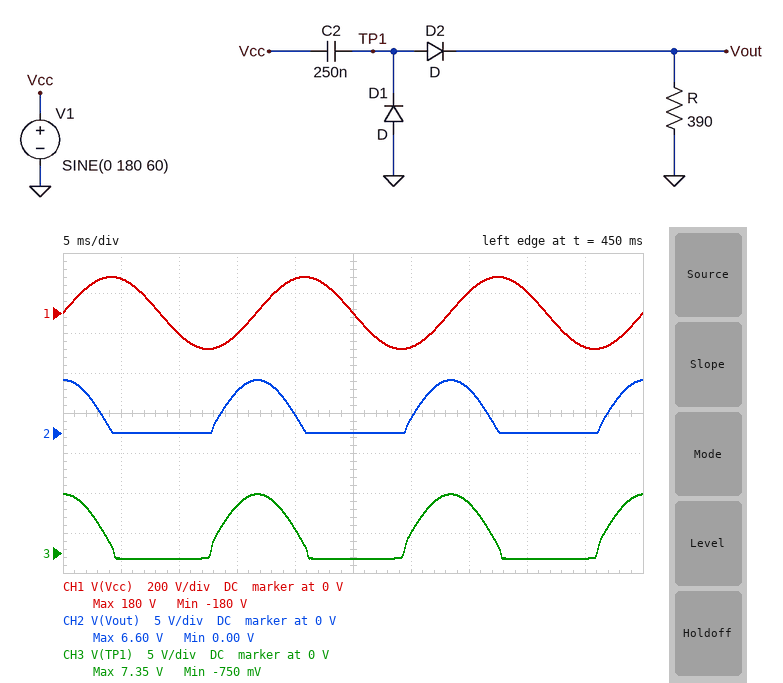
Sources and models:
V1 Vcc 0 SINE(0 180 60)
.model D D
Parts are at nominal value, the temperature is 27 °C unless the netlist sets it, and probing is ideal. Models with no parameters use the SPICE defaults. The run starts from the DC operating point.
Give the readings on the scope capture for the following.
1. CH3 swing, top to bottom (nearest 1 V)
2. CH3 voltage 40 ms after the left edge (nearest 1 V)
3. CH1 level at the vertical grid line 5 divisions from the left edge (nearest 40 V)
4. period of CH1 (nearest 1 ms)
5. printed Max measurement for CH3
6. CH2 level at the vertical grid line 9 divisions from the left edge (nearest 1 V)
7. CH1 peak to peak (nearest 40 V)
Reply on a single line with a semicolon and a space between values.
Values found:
8 V; -1 V; 0 V; 17 ms; 7.35 V; 0 V; 360 V
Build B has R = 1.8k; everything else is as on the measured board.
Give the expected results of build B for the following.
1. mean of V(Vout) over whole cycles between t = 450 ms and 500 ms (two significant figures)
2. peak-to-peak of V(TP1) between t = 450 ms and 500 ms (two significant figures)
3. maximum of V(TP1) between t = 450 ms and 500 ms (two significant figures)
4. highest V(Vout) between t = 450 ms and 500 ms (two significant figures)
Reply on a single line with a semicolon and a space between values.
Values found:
9.6 V; 32 V; 31 V; 30 V
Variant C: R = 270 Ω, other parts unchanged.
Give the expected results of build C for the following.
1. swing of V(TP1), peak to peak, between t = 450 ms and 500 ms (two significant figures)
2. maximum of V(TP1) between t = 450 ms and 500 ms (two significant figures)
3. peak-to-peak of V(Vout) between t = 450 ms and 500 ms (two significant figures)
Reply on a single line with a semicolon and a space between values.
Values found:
6.0 V; 5.3 V; 4.6 V
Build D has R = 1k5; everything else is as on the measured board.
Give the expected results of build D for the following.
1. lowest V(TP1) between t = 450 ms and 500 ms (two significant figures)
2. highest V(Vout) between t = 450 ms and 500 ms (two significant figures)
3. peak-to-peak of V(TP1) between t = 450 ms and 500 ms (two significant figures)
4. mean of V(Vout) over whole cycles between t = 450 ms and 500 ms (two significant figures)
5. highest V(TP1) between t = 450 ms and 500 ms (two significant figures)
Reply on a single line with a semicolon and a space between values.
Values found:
-730 mV; 25 V; 27 V; 8.0 V; 26 V
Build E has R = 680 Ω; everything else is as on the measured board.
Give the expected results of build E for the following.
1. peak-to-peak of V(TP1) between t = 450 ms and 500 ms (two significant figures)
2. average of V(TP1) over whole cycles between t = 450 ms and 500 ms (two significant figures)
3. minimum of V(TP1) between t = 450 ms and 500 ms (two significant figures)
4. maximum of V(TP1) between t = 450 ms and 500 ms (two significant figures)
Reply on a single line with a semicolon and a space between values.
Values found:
13 V; 3.7 V; -730 mV; 12 V
